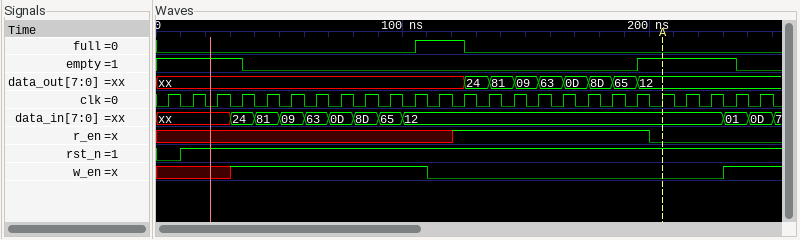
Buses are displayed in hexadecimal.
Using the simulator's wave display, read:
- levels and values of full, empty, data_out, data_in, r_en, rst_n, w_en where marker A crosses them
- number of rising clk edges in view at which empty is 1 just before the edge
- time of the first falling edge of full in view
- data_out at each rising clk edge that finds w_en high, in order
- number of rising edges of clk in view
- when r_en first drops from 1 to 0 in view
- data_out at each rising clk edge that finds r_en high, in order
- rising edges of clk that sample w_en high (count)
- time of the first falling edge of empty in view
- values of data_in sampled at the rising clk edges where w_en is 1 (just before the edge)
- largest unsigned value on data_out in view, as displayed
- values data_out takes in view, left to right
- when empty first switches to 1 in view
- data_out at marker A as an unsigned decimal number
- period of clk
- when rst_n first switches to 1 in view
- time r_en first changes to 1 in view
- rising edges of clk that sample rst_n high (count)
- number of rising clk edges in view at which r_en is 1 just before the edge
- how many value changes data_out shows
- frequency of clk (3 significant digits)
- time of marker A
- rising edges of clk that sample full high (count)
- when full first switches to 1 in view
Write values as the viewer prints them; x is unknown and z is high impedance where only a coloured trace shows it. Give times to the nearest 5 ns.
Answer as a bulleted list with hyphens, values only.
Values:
- full=0, empty=1, data_out=12, data_in=12, r_en=0, rst_n=1, w_en=0
- 8
- 125 ns
- xx, xx, xx, xx, xx, xx, xx, xx, 12, 12
- 25
- 200 ns
- xx, 24, 81, 09, 63, 0D, 8D, 65
- 10
- 35 ns
- 24, 81, 09, 63, 0D, 8D, 65, 12, 01, 0D
- 8D
- xx, 24, 81, 09, 63, 0D, 8D, 65, 12
- 195 ns
- 18
- 10 ns
- 10 ns
- 120 ns
- 24
- 8
- 8
- 100 MHz
- 205 ns
- 2
- 105 ns
